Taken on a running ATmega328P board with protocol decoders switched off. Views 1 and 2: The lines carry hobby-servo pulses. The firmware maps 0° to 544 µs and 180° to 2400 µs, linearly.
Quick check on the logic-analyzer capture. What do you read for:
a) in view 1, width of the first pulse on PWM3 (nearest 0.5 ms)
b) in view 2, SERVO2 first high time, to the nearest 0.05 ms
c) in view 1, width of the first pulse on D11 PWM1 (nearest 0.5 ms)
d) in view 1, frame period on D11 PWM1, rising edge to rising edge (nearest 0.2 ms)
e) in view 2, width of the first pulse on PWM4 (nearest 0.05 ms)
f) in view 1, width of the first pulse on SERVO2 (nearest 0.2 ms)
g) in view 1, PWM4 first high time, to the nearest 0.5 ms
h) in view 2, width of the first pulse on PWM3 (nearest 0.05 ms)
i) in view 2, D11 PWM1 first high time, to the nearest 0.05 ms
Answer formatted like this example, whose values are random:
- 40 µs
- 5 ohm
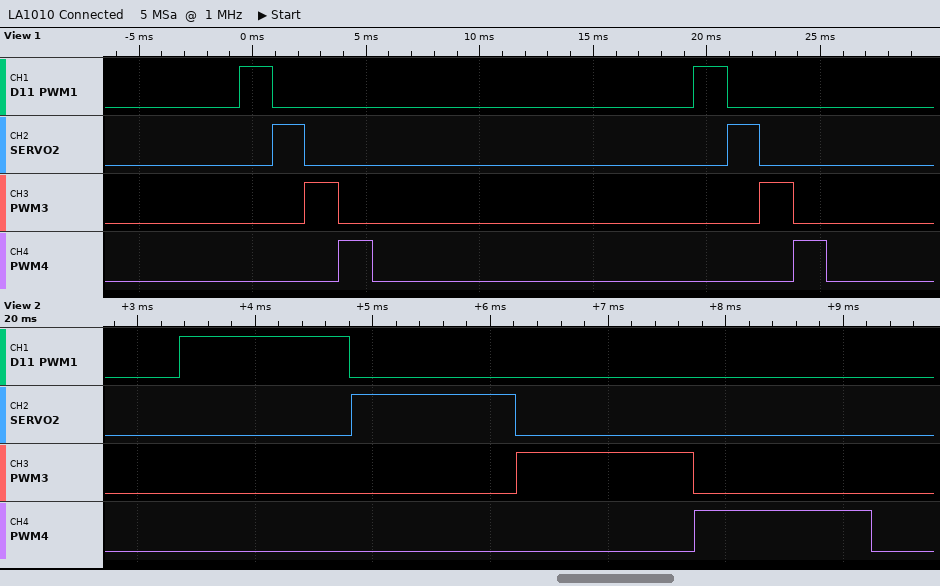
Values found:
- 1.5 ms
- 1.40 ms
- 1.5 ms
- 20.0 ms
- 1.50 ms
- 1.4 ms
- 1.5 ms
- 1.50 ms
- 1.45 ms
